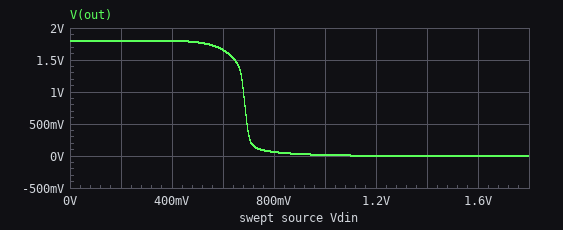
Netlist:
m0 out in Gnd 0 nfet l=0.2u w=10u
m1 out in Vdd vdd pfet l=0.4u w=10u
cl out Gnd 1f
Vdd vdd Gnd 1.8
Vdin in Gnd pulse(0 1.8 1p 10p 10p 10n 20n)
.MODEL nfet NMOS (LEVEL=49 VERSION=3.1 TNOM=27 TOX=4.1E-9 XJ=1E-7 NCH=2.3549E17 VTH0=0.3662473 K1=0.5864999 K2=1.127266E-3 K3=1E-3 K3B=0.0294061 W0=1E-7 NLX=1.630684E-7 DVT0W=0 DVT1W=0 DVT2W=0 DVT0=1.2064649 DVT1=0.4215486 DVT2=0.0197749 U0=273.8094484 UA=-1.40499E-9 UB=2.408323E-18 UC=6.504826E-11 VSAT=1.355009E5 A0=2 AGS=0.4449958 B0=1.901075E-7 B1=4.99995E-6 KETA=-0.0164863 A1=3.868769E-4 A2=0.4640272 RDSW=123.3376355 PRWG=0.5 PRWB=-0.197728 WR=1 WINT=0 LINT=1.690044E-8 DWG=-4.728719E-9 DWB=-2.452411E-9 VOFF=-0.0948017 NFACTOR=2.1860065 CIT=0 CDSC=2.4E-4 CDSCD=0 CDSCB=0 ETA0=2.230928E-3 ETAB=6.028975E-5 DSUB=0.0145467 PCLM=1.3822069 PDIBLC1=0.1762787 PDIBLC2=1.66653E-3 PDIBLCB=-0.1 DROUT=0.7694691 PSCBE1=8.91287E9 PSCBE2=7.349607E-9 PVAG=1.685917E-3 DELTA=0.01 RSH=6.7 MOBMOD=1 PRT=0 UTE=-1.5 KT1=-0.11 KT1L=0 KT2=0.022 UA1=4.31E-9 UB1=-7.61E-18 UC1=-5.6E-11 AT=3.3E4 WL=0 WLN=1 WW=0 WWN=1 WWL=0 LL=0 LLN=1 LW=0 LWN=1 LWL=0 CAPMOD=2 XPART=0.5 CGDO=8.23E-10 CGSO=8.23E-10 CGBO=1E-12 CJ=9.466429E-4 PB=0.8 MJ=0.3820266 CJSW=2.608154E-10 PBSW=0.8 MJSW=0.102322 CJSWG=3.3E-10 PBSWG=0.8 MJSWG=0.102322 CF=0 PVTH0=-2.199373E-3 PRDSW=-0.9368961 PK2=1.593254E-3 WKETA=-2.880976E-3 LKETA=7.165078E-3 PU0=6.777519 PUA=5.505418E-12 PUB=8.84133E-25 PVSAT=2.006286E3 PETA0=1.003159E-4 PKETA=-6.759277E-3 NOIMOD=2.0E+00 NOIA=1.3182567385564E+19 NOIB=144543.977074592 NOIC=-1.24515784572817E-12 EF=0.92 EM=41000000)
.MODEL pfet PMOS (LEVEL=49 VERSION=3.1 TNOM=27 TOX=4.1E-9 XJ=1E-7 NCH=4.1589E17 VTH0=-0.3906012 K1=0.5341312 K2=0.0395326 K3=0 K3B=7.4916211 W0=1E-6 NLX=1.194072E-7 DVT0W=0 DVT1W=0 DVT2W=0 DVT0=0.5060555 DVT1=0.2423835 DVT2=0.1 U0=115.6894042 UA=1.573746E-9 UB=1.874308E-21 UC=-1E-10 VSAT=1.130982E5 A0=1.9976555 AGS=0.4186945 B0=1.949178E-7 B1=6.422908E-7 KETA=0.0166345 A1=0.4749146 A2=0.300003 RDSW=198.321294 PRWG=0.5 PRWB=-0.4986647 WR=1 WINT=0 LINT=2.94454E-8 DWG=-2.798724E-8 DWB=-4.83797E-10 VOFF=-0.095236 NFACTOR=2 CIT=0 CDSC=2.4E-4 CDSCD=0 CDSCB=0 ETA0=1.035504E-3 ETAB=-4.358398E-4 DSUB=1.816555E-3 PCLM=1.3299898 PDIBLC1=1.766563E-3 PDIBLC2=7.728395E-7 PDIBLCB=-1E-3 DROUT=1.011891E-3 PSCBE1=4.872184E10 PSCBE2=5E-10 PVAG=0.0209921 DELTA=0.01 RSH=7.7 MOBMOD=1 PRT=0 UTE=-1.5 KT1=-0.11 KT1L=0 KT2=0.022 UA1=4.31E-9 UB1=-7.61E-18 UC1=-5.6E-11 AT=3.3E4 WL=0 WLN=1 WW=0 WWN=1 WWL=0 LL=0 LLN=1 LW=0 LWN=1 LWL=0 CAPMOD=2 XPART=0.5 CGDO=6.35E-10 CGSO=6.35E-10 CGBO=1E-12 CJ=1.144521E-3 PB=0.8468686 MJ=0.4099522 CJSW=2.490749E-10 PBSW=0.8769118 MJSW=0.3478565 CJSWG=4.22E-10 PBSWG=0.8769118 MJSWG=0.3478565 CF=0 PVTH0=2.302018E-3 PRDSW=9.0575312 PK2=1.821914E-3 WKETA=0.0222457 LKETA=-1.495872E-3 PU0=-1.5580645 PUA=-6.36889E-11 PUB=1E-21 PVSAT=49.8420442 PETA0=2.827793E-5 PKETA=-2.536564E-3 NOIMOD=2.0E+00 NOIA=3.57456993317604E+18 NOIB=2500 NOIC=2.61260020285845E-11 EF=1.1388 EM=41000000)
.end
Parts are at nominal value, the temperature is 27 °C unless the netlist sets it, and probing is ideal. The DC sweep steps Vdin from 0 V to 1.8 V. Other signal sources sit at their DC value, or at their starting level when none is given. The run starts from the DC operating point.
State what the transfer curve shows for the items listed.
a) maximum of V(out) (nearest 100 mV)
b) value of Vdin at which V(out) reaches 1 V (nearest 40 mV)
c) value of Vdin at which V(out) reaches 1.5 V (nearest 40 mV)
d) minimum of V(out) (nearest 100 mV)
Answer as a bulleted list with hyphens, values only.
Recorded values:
- 1.8 V
- 680 mV
- 640 mV
- 0 V
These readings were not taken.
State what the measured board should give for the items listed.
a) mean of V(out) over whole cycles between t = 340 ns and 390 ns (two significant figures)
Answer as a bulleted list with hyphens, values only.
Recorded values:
- 900 mV
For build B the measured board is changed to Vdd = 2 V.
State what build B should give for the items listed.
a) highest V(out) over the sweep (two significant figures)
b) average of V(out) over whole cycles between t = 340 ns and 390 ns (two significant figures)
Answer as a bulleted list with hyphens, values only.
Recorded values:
- 2.0 V
- 1.0 V
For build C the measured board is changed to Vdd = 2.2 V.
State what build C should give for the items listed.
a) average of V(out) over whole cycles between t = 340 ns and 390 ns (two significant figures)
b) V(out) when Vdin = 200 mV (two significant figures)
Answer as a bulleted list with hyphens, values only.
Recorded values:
- 1.1 V
- 2.2 V
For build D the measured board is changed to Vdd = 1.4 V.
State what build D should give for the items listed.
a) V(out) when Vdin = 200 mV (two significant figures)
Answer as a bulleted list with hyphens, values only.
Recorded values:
- 1.4 V
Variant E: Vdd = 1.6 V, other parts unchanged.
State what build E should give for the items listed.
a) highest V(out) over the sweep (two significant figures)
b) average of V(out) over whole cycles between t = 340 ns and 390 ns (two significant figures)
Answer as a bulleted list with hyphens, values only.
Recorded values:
- 1.6 V
- 800 mV
